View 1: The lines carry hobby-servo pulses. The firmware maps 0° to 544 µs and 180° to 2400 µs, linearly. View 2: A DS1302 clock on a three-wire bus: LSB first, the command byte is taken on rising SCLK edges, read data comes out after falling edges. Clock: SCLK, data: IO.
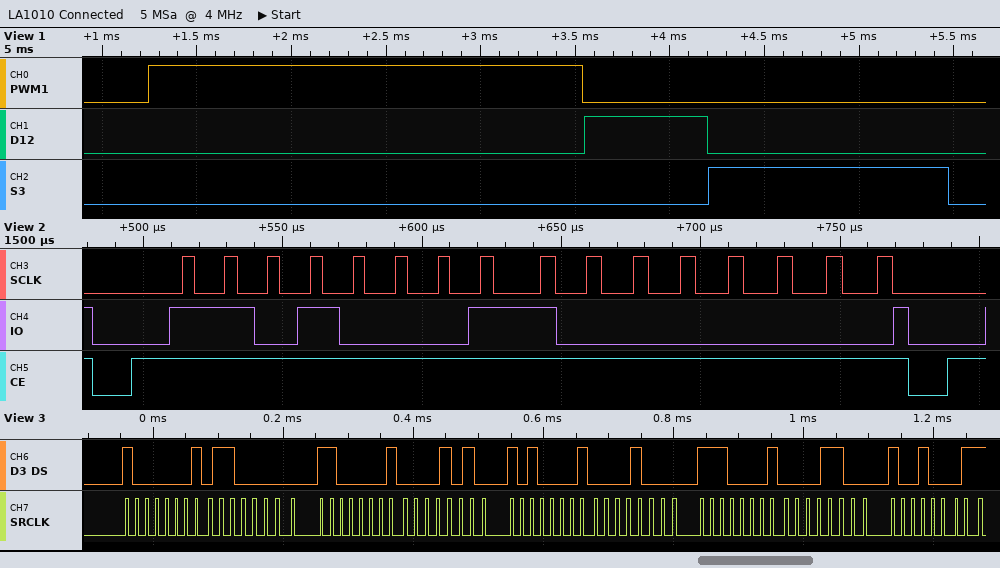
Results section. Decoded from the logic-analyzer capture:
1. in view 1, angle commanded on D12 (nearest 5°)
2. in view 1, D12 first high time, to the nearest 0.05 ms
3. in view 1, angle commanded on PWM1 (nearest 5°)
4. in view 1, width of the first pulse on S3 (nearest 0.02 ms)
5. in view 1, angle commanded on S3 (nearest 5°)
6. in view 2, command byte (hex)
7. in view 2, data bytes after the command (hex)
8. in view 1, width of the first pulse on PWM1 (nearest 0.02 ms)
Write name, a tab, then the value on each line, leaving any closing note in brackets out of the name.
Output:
in view 1, angle commanded on D12	10°
in view 1, D12 first high time, to the nearest 0.05 ms	0.65 ms
in view 1, angle commanded on PWM1	170°
in view 1, width of the first pulse on S3	1.26 ms
in view 1, angle commanded on S3	70°
in view 2, command byte	0x8B
in view 2, data bytes after the command	01
in view 1, width of the first pulse on PWM1	2.30 ms
